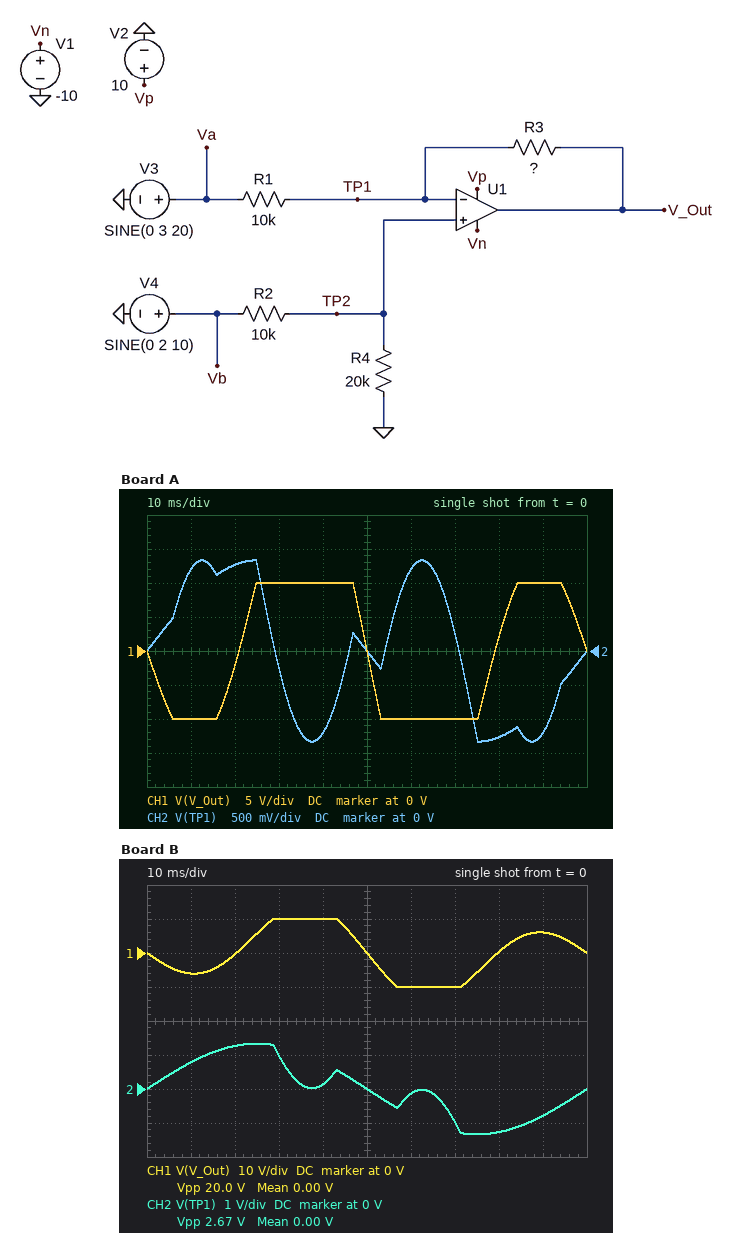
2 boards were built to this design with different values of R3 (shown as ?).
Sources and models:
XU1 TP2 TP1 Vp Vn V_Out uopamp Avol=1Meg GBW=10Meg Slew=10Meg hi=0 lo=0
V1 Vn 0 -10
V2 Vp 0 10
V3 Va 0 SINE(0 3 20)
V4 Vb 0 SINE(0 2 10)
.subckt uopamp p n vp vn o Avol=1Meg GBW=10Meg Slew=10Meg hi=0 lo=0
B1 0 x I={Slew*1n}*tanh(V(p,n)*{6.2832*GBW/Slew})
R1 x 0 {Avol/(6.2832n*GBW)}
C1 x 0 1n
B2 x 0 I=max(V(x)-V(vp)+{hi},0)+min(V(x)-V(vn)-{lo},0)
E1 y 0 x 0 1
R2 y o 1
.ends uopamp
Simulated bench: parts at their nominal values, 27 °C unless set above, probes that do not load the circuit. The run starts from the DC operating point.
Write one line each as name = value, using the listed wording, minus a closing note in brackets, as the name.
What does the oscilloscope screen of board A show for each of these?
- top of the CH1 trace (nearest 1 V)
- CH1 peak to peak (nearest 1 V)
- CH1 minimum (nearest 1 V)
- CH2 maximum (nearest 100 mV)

top of the CH1 trace = 10 V
CH1 peak to peak = 20 V
CH1 minimum = -10 V
CH2 maximum = 1.3 V
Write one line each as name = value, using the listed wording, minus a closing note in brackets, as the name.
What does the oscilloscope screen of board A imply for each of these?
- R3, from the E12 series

R3, from the E12 series = 68 kΩ
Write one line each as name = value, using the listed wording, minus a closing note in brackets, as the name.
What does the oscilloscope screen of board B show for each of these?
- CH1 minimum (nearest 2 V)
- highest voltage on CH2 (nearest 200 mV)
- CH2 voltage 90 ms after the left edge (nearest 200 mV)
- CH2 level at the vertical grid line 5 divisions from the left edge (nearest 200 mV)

CH1 minimum = -10 V
highest voltage on CH2 = 1.4 V
CH2 voltage 90 ms after the left edge = -800 mV
CH2 level at the vertical grid line 5 divisions from the left edge = 0 V
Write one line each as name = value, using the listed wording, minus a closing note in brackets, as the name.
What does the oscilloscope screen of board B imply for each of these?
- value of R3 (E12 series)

value of R3 = 33 kΩ
